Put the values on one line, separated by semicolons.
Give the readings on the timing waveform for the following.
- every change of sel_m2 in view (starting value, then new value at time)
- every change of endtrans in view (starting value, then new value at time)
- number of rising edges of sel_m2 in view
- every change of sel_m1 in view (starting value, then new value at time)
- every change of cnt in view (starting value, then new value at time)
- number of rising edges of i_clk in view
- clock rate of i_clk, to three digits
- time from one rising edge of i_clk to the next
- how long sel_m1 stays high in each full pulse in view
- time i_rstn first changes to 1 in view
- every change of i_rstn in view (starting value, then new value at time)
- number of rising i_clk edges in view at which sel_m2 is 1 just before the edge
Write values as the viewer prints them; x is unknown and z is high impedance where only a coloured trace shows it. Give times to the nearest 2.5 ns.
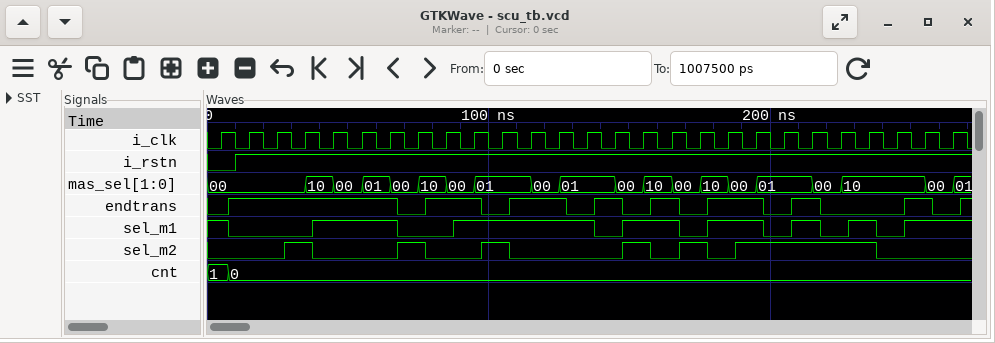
0, 1 at 27.5 ns, 0 at 37.5 ns, 1 at 67.5 ns, 0 at 77.5 ns, 1 at 97.5 ns, 0 at 107.5 ns, 1 at 147.5 ns, 0 at 157.5 ns, 1 at 167.5 ns, 0 at 177.5 ns, 1 at 187.5 ns, 0 at 237.5 ns; 0, 1 at 7.5 ns, 0 at 67.5 ns, 1 at 77.5 ns, 0 at 97.5 ns, 1 at 107.5 ns, 0 at 127.5 ns, 1 at 137.5 ns, 0 at 147.5 ns, 1 at 157.5 ns, 0 at 167.5 ns, 1 at 177.5 ns, 0 at 197.5 ns, 1 at 207.5 ns, 0 at 217.5 ns, 1 at 247.5 ns, 0 at 257.5 ns, 1 at 267.5 ns; 6; 1, 0 at 7.5 ns, 1 at 37.5 ns, 0 at 67.5 ns, 1 at 87.5 ns, 0 at 137.5 ns, 1 at 147.5 ns, 0 at 167.5 ns, 1 at 177.5 ns, 0 at 197.5 ns, 1 at 207.5 ns, 0 at 217.5 ns, 1 at 227.5 ns, 0 at 237.5 ns, 1 at 247.5 ns; 1, 0 at 7.5 ns; 27; 100 MHz; 10 ns; 30 ns, 50 ns, 20 ns, 20 ns, 10 ns, 10 ns; 10 ns; 0, 1 at 10 ns; 10
